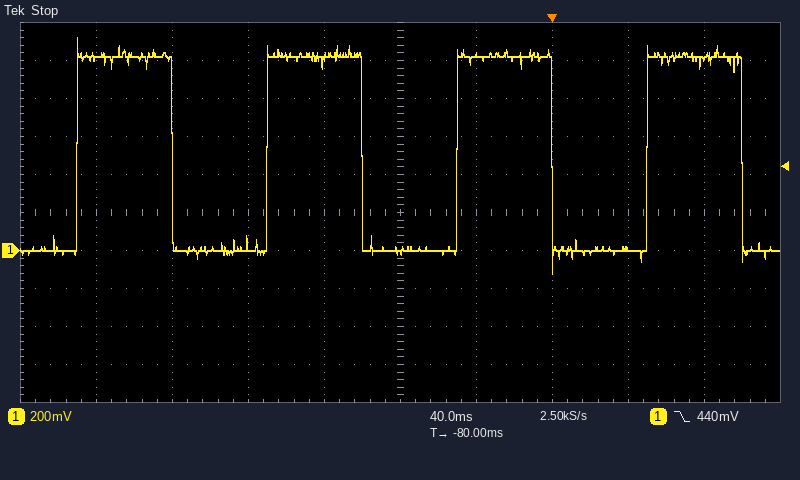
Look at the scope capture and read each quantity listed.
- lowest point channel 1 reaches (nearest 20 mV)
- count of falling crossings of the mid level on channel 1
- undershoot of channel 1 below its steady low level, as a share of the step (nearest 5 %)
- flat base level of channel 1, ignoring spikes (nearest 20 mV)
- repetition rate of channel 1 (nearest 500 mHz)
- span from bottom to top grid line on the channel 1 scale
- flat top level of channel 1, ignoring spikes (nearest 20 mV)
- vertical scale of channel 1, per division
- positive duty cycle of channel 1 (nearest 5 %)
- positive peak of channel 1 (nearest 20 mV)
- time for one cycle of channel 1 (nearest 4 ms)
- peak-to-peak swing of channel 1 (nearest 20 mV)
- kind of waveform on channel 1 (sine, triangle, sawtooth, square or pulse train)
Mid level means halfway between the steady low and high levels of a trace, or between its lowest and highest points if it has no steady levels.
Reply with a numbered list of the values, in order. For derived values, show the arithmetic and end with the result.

1. -120 mV
2. 4
3. 10 %
4. 0 mV
5. 1 / 100 ms ≈ 10.0 Hz
6. 2 V
7. 1.02 V
8. 200 mV
9. 50 %
10. 1.12 V
11. 100 ms
12. 1.12 V − (-120 mV) = 1.24 V
13. square
